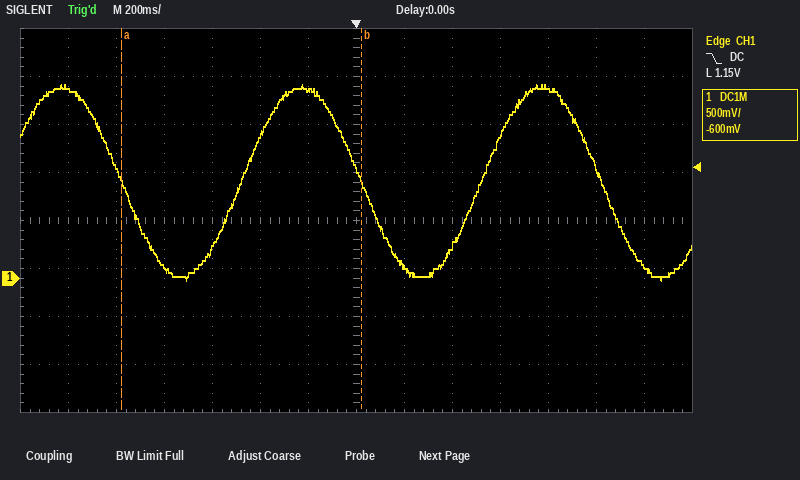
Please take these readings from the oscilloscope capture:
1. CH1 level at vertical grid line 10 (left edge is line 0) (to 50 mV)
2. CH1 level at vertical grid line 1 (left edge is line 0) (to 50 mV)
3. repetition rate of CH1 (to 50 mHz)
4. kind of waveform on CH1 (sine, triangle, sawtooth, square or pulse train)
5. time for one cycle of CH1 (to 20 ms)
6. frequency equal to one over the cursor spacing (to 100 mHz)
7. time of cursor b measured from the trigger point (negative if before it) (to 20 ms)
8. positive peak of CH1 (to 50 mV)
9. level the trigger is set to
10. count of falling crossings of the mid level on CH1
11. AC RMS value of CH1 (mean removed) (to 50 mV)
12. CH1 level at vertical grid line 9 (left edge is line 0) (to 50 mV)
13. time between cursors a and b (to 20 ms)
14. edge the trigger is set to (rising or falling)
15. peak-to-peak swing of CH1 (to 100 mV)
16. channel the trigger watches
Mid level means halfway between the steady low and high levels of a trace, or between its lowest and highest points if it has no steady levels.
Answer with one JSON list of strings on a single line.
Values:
["1.50 V", "1.95 V", "1.00 Hz", "sine", "1.00 s", "1.0 Hz", "+20 ms", "2.00 V", "1.15 V", "3", "700 mV", "350 mV", "1.00 s", "falling", "2.00 V", "CH1"]
